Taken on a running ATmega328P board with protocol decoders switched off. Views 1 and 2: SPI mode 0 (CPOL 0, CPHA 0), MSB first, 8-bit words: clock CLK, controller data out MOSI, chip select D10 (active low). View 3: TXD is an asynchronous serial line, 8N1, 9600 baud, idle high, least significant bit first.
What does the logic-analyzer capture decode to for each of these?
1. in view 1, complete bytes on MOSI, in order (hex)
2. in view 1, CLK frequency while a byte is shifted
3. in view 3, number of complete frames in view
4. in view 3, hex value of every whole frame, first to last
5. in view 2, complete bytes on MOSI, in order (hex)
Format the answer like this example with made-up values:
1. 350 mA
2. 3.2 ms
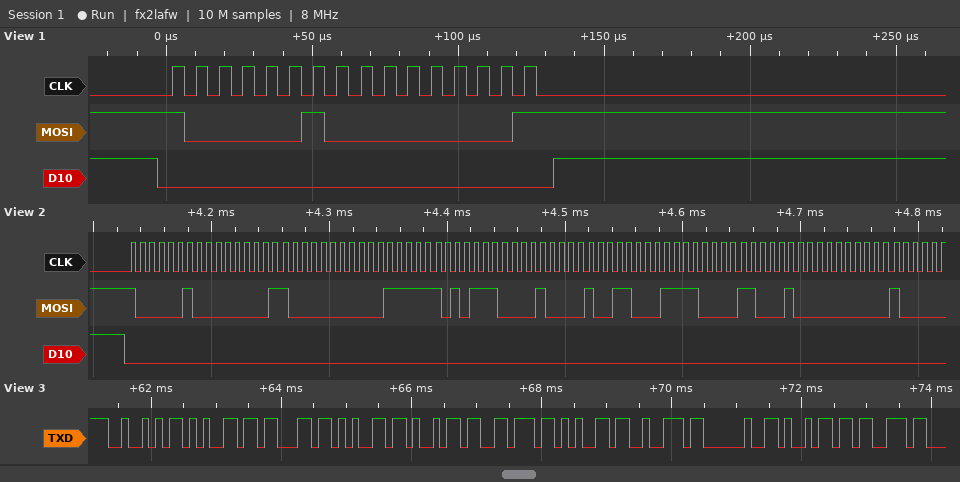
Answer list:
1. 82 01
2. 125 kHz
3. 11
4. 0x52 0x65 0x63 0x65 0x69 0x76 0x65 0x72 0x20 0x69 0x73
5. 82 01 80 1F AE 10 98 F0 C4 00
